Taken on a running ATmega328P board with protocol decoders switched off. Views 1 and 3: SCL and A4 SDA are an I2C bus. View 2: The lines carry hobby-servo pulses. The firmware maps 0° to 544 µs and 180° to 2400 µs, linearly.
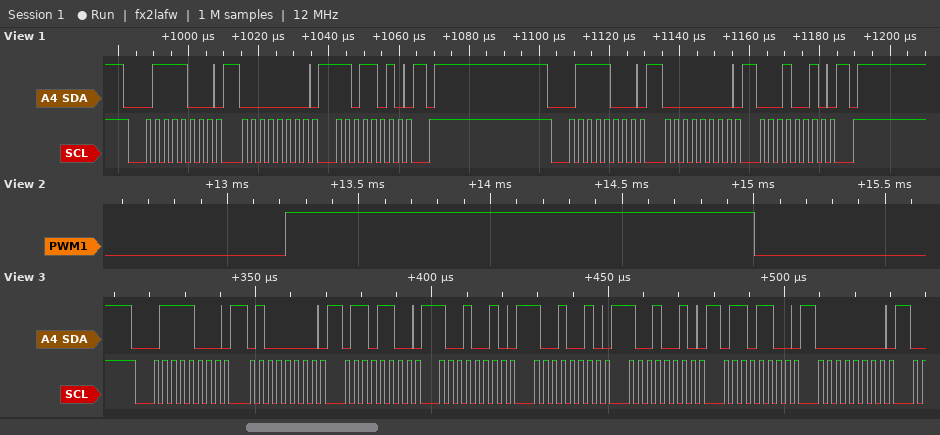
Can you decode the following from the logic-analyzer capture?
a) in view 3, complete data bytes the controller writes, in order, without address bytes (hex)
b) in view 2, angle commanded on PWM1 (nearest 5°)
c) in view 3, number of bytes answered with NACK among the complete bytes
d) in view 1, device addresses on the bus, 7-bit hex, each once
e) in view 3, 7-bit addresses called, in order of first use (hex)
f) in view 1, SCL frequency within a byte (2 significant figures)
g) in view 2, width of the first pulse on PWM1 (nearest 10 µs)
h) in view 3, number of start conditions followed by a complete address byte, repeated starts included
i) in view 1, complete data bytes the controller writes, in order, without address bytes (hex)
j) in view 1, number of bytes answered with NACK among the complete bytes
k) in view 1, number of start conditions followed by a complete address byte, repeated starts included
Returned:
40 6C 92 92 92 6C 00
120°
0
0x3C
0x3C
400 kHz
1780 µs
1
00 DA 00 12
0
2
